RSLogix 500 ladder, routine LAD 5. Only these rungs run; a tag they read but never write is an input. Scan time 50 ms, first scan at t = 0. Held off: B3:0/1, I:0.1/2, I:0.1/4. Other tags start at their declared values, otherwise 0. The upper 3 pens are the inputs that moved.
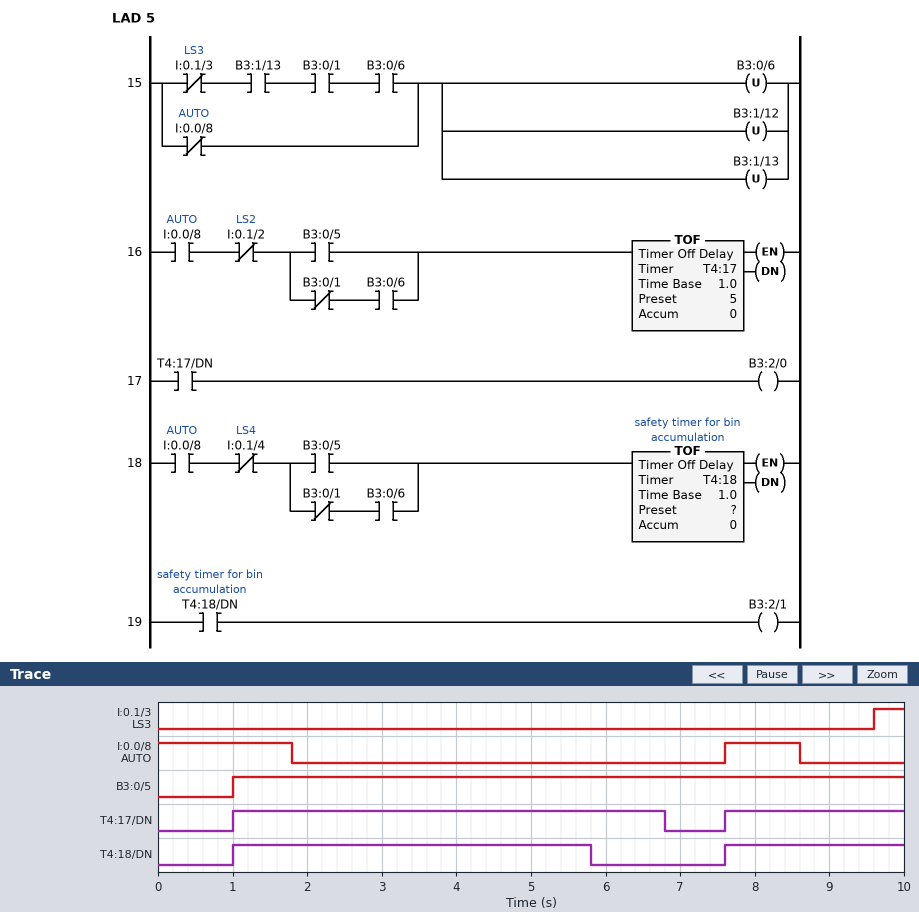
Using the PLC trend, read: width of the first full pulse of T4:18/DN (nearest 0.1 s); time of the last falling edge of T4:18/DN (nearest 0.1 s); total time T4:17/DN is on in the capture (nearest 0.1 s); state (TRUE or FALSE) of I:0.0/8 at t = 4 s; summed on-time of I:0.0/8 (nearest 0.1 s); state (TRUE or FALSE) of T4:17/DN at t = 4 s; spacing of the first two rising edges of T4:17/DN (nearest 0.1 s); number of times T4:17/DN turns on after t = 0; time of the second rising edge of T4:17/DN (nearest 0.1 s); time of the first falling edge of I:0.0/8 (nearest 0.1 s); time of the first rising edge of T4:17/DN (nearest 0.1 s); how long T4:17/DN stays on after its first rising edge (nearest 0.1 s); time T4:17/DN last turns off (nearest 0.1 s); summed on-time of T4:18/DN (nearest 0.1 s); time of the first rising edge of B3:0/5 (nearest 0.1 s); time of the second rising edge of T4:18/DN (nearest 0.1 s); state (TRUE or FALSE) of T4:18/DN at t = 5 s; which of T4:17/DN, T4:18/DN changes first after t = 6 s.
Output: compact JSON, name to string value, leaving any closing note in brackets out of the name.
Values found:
{"width of the first full pulse of T4:18/DN": "4.8 s", "time of the last falling edge of T4:18/DN": "5.8 s", "total time T4:17/DN is on in the capture": "8.2 s", "state (TRUE or FALSE) of I:0.0/8 at t = 4 s": "FALSE", "summed on-time of I:0.0/8": "2.8 s", "state (TRUE or FALSE) of T4:17/DN at t = 4 s": "TRUE", "spacing of the first two rising edges of T4:17/DN": "6.6 s", "number of times T4:17/DN turns on after t = 0": "2", "time of the second rising edge of T4:17/DN": "7.6 s", "time of the first falling edge of I:0.0/8": "1.8 s", "time of the first rising edge of T4:17/DN": "1.0 s", "how long T4:17/DN stays on after its first rising edge": "5.8 s", "time T4:17/DN last turns off": "6.8 s", "summed on-time of T4:18/DN": "7.2 s", "time of the first rising edge of B3:0/5": "1.0 s", "time of the second rising edge of T4:18/DN": "7.6 s", "state (TRUE or FALSE) of T4:18/DN at t = 5 s": "TRUE", "which of T4:17/DN, T4:18/DN changes first after t = 6 s": "T4:17/DN"}
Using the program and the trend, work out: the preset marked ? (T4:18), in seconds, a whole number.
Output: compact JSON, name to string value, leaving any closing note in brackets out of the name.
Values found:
{"the preset marked ? (T4:18), in seconds, a whole number": "4 s"}
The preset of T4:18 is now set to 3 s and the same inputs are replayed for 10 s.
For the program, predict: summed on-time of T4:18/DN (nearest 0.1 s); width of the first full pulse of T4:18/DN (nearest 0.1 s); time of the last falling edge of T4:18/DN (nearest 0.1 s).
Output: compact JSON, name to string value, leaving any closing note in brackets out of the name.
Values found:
{"summed on-time of T4:18/DN": "6.2 s", "width of the first full pulse of T4:18/DN": "3.8 s", "time of the last falling edge of T4:18/DN": "4.8 s"}
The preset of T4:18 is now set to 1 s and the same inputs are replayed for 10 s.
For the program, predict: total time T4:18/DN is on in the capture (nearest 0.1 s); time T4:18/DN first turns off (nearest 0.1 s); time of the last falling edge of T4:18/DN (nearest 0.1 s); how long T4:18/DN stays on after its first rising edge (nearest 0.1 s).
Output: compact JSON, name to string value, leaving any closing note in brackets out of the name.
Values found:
{"total time T4:18/DN is on in the capture": "3.8 s", "time T4:18/DN first turns off": "2.8 s", "time of the last falling edge of T4:18/DN": "9.6 s", "how long T4:18/DN stays on after its first rising edge": "1.8 s"}
